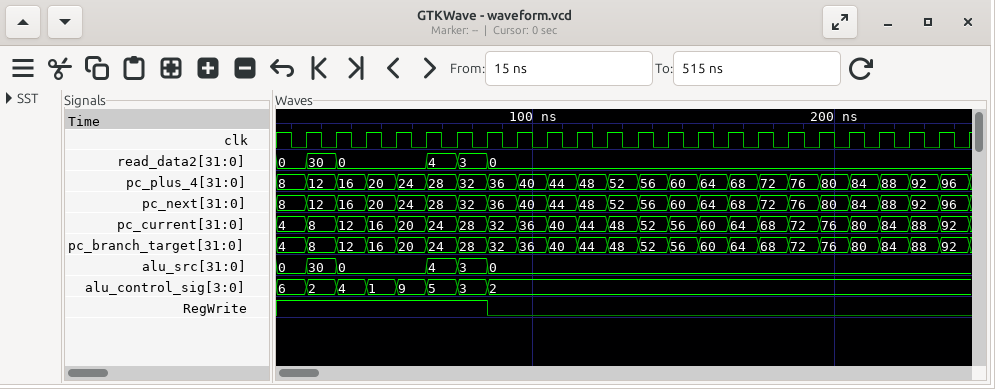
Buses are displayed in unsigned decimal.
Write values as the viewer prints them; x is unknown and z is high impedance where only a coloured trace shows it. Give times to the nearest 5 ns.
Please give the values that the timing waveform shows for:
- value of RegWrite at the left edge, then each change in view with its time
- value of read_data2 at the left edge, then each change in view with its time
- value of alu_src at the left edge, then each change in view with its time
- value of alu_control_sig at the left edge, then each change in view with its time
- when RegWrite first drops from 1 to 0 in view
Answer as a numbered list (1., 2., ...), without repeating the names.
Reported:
1. 1, 0 at 85 ns
2. 0, 30 at 25 ns, 0 at 35 ns, 4 at 65 ns, 3 at 75 ns, 0 at 85 ns
3. 0, 30 at 25 ns, 0 at 35 ns, 4 at 65 ns, 3 at 75 ns, 0 at 85 ns
4. 6, 2 at 25 ns, 4 at 35 ns, 1 at 45 ns, 9 at 55 ns, 5 at 65 ns, 3 at 75 ns, 2 at 85 ns
5. 85 ns
